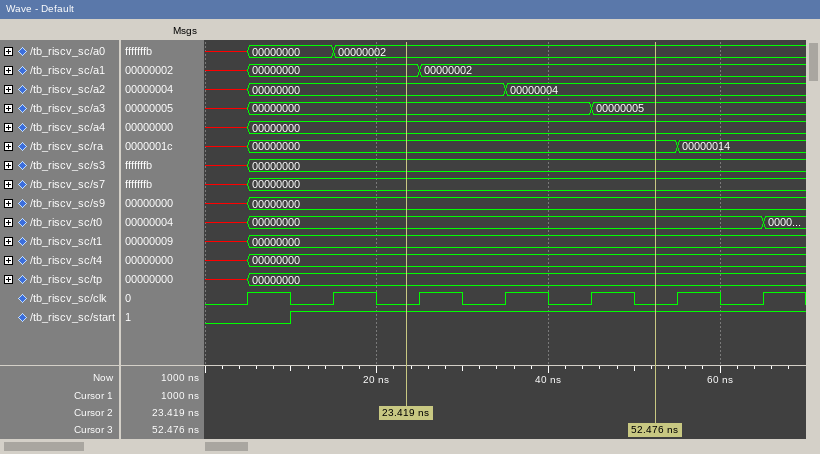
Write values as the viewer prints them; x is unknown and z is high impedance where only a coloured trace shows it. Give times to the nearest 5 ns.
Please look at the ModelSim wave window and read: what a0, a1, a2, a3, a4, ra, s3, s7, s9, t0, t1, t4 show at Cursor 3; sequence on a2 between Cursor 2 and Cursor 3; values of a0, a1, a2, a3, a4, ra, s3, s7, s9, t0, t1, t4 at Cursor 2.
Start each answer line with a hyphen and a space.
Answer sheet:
- a0=00000002, a1=00000002, a2=00000004, a3=00000005, a4=00000000, ra=00000000, s3=00000000, s7=00000000, s9=00000000, t0=00000000, t1=00000000, t4=00000000
- 00000000, 00000004
- a0=00000002, a1=00000000, a2=00000000, a3=00000000, a4=00000000, ra=00000000, s3=00000000, s7=00000000, s9=00000000, t0=00000000, t1=00000000, t4=00000000
